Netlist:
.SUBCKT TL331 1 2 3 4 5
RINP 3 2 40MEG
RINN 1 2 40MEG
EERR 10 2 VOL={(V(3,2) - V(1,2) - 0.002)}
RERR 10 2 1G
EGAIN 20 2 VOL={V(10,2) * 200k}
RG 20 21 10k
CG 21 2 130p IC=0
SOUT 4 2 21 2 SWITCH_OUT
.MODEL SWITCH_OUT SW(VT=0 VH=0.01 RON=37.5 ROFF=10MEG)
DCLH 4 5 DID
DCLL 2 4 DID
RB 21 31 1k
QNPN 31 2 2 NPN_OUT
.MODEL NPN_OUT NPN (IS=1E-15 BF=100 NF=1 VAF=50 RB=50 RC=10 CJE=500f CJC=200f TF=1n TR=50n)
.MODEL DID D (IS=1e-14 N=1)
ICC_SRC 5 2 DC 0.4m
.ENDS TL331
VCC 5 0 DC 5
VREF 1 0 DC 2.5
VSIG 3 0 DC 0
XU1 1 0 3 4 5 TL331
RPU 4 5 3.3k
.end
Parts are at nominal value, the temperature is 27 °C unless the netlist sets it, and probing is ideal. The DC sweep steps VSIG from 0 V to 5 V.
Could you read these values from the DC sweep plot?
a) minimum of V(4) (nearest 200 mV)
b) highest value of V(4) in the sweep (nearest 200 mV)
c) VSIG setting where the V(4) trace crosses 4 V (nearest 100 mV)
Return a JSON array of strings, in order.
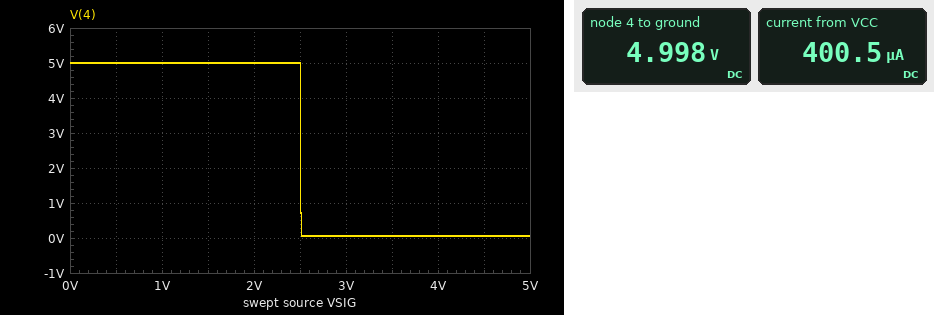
["0 V", "5.0 V", "2.5 V"]
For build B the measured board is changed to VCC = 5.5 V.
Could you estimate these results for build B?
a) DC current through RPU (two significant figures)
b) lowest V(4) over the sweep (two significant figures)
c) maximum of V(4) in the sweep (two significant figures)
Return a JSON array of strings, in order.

["550 nA", "62 mV", "5.5 V"]
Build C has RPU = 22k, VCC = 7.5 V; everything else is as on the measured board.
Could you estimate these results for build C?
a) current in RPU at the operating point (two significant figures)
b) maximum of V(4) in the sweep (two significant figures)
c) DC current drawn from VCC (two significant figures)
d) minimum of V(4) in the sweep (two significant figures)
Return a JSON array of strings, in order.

["750 nA", "7.5 V", "400 µA", "13 mV"]
